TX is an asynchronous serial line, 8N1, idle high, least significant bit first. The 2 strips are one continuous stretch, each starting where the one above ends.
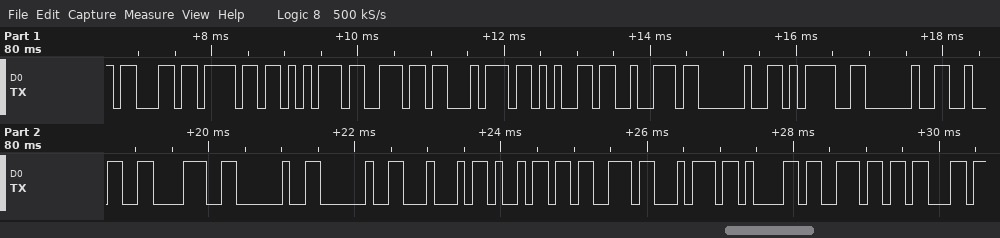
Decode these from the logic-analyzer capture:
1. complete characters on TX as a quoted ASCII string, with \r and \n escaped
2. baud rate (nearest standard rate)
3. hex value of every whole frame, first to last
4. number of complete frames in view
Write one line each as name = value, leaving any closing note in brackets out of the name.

complete characters on TX as a quoted ASCII string, with \r and \n escaped = "counter = 28  Distanc"
baud rate = 9600 baud
hex value of every whole frame, first to last = 63 6F 75 6E 74 65 72 20 3D 20 32 38 20 20 44 69 73 74 61 6E 63
number of complete frames in view = 21
